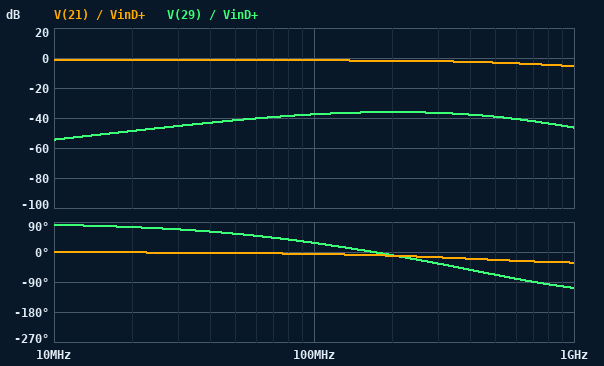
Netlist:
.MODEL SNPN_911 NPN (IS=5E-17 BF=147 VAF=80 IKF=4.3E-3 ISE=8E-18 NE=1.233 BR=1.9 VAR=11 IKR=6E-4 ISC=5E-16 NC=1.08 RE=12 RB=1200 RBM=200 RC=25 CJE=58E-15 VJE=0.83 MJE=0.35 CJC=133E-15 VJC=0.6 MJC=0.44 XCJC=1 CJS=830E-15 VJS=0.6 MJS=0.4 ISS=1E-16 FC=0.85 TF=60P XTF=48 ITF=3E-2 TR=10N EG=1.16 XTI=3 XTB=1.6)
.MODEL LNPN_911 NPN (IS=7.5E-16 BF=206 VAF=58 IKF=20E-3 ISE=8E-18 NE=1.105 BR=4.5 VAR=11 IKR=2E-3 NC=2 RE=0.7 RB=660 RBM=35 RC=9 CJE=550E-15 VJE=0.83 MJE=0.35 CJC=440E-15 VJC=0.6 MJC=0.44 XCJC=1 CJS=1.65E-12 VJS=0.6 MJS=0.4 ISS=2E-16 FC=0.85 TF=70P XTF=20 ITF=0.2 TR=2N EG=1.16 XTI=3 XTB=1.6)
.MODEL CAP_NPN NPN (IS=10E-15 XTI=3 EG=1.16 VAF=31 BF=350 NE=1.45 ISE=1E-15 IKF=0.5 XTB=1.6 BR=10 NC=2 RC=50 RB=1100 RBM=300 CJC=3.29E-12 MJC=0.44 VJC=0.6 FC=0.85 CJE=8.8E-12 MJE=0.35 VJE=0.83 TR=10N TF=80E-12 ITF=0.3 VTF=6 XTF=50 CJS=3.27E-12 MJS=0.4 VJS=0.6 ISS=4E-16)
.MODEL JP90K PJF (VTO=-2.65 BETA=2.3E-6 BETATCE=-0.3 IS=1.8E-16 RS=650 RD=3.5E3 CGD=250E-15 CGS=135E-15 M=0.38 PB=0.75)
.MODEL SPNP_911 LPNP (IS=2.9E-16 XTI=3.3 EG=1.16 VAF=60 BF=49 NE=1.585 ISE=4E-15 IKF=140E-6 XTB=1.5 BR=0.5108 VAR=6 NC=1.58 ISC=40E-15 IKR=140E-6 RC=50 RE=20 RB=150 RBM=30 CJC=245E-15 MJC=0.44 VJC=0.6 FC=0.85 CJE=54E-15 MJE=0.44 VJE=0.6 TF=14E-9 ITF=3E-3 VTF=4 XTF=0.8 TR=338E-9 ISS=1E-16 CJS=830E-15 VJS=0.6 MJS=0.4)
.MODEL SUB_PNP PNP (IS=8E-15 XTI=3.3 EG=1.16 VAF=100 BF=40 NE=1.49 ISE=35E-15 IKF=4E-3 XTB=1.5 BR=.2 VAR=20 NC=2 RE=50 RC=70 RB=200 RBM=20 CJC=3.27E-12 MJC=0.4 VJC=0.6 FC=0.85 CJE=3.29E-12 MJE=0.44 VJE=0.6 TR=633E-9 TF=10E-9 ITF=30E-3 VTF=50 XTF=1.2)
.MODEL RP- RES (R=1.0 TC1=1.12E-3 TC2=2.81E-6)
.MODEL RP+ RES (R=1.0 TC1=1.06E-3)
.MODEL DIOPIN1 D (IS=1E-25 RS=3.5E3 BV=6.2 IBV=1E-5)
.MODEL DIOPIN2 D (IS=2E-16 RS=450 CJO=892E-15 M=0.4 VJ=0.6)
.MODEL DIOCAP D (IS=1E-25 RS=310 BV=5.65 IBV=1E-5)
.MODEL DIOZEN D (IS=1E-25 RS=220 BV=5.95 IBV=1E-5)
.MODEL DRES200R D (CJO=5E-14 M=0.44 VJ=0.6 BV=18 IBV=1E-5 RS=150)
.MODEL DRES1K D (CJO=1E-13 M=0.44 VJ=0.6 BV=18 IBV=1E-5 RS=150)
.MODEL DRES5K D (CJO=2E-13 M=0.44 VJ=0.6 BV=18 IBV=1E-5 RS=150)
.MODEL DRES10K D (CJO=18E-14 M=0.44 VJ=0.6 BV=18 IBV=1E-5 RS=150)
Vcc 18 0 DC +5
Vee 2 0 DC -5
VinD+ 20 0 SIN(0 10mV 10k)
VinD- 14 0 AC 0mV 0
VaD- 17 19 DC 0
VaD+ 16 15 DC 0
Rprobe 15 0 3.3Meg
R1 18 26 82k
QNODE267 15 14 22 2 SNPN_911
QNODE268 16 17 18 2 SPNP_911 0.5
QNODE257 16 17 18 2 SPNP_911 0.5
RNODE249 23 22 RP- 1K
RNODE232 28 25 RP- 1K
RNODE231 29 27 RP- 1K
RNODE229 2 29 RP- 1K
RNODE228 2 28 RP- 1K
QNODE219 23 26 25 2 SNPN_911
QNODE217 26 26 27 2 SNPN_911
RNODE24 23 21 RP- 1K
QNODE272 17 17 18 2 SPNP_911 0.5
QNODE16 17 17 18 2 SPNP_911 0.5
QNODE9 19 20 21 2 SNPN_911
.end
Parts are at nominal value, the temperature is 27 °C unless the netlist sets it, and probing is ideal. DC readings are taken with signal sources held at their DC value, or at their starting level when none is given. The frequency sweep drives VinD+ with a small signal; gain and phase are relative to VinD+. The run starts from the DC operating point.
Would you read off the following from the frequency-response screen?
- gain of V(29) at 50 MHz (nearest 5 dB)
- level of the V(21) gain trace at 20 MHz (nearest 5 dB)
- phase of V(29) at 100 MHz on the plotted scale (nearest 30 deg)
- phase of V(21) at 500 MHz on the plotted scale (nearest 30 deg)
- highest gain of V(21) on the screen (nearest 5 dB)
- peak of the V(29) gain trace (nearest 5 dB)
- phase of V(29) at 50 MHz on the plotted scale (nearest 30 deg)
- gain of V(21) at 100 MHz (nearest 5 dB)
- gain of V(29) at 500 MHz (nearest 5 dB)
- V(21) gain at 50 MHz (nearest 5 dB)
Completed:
-40 dB
0 dB
30 deg
-30 deg
0 dB
-35 dB
60 deg
0 dB
-40 dB
0 dB
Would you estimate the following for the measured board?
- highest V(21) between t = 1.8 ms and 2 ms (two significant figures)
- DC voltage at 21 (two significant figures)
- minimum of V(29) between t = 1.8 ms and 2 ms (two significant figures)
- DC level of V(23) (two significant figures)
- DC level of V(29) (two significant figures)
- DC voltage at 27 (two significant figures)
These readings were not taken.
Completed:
-710 mV
-720 mV
-4.9 V
-770 mV
-4.9 V
-4.8 V
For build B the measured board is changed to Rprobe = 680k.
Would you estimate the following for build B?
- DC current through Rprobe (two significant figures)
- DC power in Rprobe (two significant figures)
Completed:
860 nA
510 nW
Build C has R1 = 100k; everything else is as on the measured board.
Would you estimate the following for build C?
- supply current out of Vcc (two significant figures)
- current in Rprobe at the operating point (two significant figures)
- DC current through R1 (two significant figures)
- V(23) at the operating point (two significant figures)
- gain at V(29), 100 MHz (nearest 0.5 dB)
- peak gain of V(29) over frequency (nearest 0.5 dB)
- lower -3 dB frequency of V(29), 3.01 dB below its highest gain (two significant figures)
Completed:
180 µA
360 nA
91 µA
-760 mV
-38.0 dB
-36.5 dB
70 MHz
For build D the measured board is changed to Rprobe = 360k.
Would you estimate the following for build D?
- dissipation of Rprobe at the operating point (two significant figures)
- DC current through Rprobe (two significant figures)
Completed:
430 nW
1.1 µA
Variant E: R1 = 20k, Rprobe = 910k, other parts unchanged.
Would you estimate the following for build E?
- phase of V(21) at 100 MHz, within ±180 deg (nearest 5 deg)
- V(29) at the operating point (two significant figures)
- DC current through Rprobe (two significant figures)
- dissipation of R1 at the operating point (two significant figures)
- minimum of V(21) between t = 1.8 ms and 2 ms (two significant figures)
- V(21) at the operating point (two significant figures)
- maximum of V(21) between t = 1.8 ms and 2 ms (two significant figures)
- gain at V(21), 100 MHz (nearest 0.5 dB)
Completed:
-5 deg
-4.6 V
670 nA
3.5 mW
-770 mV
-760 mV
-750 mV
-0.5 dB
